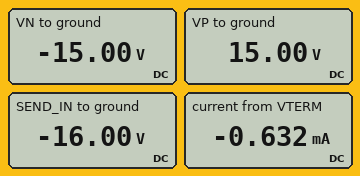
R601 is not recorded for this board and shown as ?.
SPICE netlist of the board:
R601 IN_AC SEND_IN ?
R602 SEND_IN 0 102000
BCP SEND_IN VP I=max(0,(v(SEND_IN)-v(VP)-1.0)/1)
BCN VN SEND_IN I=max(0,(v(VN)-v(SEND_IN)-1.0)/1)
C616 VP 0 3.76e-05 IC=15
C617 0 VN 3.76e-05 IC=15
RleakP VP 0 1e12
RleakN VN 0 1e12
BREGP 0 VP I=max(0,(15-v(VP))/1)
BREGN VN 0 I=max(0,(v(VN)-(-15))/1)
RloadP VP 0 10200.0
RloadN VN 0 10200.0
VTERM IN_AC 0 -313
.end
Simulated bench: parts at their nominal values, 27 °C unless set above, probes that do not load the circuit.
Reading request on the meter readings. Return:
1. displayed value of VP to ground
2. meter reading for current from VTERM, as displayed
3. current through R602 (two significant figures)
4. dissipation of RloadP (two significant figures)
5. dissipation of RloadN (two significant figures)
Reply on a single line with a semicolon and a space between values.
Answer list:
15.00 V; -0.632 mA; 160 µA; 22 mW; 22 mW
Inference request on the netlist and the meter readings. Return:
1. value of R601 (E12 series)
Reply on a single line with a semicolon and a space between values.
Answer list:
470 kΩ
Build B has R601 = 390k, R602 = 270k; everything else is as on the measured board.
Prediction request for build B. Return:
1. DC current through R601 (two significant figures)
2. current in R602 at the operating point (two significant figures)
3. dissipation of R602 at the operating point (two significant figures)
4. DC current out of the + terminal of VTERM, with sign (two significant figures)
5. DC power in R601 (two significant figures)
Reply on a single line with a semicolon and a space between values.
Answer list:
760 µA; 59 µA; 950 µW; -760 µA; 230 mW
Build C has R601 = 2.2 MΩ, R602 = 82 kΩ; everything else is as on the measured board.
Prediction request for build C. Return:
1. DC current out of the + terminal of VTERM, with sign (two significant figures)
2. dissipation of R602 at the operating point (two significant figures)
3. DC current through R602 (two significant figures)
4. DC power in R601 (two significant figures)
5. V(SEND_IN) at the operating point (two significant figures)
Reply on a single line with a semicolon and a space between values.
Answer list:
-140 µA; 1.5 mW; 140 µA; 41 mW; -11 V
